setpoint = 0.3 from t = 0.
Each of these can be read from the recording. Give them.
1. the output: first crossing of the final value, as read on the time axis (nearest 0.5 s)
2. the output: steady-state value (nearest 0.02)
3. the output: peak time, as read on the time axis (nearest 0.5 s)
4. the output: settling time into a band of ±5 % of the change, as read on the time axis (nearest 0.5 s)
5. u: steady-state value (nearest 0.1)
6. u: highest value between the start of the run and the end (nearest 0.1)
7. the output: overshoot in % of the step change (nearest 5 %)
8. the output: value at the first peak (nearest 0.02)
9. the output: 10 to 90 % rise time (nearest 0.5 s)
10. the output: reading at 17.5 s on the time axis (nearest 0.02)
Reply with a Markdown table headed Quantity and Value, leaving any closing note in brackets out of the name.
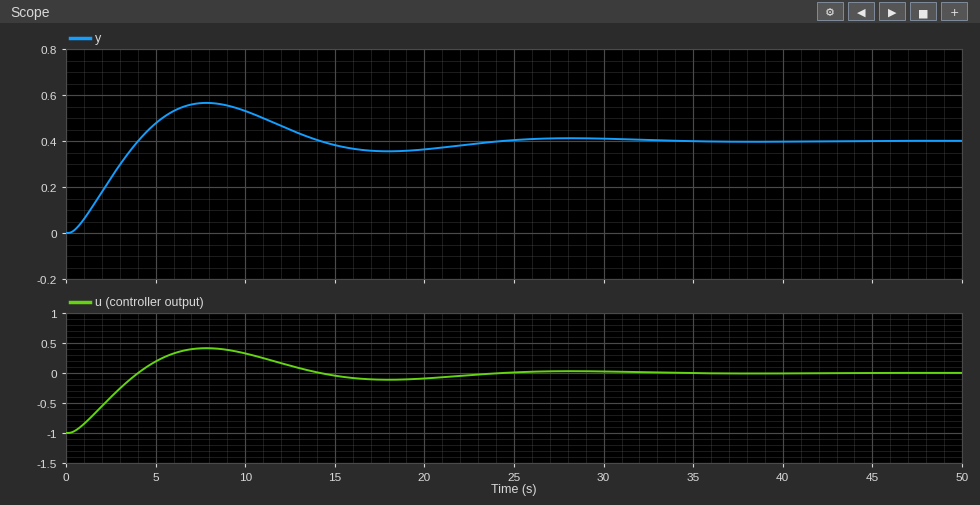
| Quantity | Value |
|---|---|
| the output: first crossing of the final value, as read on the time axis | 4.0 s |
| the output: steady-state value | 0.40 |
| the output: peak time, as read on the time axis | 8.0 s |
| the output: settling time into a band of ±5 % of the change, as read on the time axis | 22.0 s |
| u: steady-state value | 0.0 |
| u: highest value between the start of the run and the end | 0.4 |
| the output: overshoot in % of the step change | 40 % |
| the output: value at the first peak | 0.56 |
| the output: 10 to 90 % rise time | 3.0 s |
| the output: reading at 17.5 s on the time axis | 0.36 |
